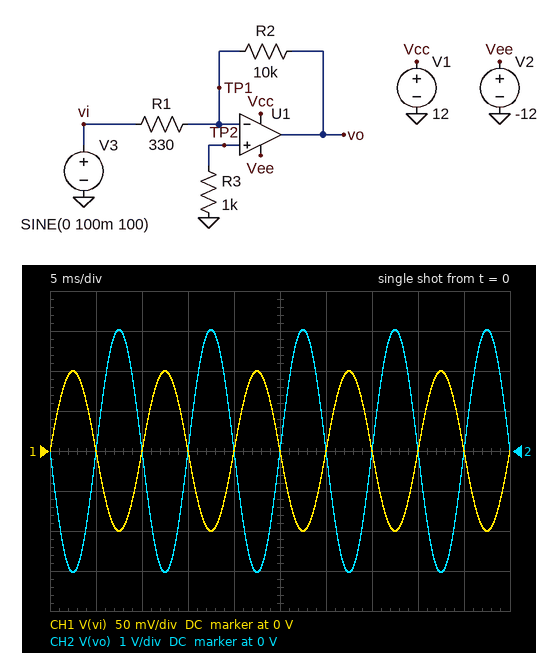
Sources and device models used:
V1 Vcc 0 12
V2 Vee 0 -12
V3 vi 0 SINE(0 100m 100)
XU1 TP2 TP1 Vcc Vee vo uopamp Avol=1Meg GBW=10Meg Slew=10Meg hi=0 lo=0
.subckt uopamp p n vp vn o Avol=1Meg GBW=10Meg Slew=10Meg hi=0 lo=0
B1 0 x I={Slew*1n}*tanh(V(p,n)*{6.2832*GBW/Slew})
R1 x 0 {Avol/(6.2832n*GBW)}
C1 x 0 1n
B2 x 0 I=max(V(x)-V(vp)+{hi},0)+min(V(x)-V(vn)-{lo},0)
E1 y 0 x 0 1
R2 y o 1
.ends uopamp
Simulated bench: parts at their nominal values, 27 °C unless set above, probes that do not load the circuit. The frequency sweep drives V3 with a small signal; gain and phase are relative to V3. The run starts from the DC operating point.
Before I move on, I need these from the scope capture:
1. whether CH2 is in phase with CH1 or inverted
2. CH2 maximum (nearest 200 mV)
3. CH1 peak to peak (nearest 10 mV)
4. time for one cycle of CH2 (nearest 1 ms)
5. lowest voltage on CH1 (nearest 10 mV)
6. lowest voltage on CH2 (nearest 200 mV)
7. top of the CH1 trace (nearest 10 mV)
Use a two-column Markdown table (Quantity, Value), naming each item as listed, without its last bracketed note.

| Quantity | Value |
|---|---|
| whether CH2 is in phase with CH1 or inverted | inverted |
| CH2 maximum | 3.0 V |
| CH1 peak to peak | 200 mV |
| time for one cycle of CH2 | 10 ms |
| lowest voltage on CH1 | -100 mV |
| lowest voltage on CH2 | -3.0 V |
| top of the CH1 trace | 100 mV |
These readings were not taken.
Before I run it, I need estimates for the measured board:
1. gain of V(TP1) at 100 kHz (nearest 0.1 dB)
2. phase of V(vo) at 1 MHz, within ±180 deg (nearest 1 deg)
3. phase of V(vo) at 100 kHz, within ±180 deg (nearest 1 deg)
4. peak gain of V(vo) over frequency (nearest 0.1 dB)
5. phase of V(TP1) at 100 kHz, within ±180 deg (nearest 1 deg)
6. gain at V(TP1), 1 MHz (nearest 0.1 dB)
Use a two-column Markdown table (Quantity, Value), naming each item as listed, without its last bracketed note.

| Quantity | Value |
|---|---|
| gain of V(TP1) at 100 kHz | -10.8 dB |
| phase of V(vo) at 1 MHz, within ±180 deg | 108 deg |
| phase of V(vo) at 100 kHz, within ±180 deg | 163 deg |
| peak gain of V(vo) over frequency | 29.6 dB |
| phase of V(TP1) at 100 kHz, within ±180 deg | 73 deg |
| gain at V(TP1), 1 MHz | -0.7 dB |
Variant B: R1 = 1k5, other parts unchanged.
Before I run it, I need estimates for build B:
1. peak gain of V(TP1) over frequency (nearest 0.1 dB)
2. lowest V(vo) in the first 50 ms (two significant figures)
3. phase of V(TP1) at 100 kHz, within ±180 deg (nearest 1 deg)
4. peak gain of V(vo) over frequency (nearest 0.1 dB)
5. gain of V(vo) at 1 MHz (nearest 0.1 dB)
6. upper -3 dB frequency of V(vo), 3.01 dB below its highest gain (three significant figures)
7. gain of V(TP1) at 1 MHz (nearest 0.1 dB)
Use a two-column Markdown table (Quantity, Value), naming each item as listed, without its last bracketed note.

| Quantity | Value |
|---|---|
| peak gain of V(TP1) over frequency | -1.2 dB |
| lowest V(vo) in the first 50 ms | -670 mV |
| phase of V(TP1) at 100 kHz, within ±180 deg | 86 deg |
| peak gain of V(vo) over frequency | 16.5 dB |
| gain of V(vo) at 1 MHz | 14.5 dB |
| upper -3 dB frequency of V(vo), 3.01 dB below its highest gain | 1.30 MHz |
| gain of V(TP1) at 1 MHz | -5.5 dB |
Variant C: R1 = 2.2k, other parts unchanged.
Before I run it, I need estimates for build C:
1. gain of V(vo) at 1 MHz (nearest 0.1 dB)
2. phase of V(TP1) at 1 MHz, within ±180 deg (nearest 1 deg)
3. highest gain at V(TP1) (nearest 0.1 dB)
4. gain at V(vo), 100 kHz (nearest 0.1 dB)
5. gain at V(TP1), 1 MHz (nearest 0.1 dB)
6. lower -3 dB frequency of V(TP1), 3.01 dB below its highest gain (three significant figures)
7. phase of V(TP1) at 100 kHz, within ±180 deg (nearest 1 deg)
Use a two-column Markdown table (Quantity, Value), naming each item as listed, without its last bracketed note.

| Quantity | Value |
|---|---|
| gain of V(vo) at 1 MHz | 12.0 dB |
| phase of V(TP1) at 1 MHz, within ±180 deg | 61 deg |
| highest gain at V(TP1) | -1.7 dB |
| gain at V(vo), 100 kHz | 13.1 dB |
| gain at V(TP1), 1 MHz | -8.0 dB |
| lower -3 dB frequency of V(TP1), 3.01 dB below its highest gain | 1.80 MHz |
| phase of V(TP1) at 100 kHz, within ±180 deg | 87 deg |
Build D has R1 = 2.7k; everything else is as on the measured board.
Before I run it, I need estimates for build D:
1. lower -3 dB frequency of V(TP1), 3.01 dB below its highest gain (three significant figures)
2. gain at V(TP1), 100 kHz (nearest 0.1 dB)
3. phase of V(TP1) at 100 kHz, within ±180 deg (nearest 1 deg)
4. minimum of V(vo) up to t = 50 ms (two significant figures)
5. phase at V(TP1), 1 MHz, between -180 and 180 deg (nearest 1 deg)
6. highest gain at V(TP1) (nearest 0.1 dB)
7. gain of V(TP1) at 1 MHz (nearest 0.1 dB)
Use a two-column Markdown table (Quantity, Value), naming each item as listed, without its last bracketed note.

| Quantity | Value |
|---|---|
| lower -3 dB frequency of V(TP1), 3.01 dB below its highest gain | 2.13 MHz |
| gain at V(TP1), 100 kHz | -28.6 dB |
| phase of V(TP1) at 100 kHz, within ±180 deg | 87 deg |
| minimum of V(vo) up to t = 50 ms | -370 mV |
| phase at V(TP1), 1 MHz, between -180 and 180 deg | 65 deg |
| highest gain at V(TP1) | -2.1 dB |
| gain of V(TP1) at 1 MHz | -9.5 dB |
